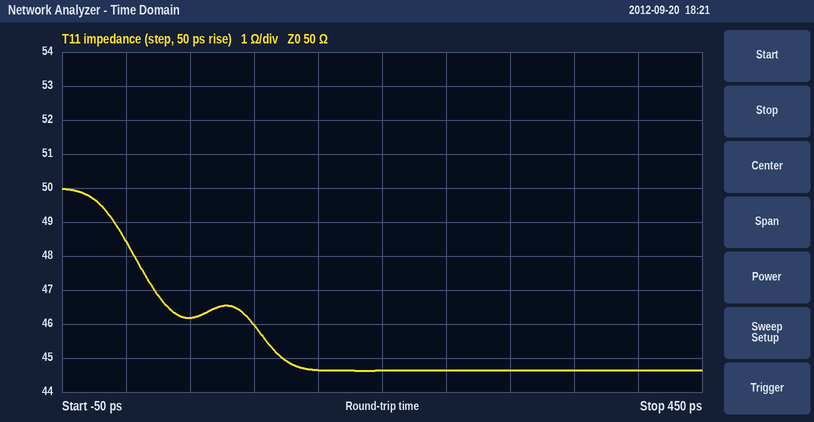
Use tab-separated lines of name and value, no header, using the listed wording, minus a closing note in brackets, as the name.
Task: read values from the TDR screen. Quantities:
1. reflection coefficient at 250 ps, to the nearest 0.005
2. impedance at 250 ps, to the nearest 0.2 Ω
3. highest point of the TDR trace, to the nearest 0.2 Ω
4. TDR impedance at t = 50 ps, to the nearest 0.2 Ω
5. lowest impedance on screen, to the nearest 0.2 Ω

reflection coefficient at 250 ps, to the nearest 0.005	-0.055
impedance at 250 ps, to the nearest 0.2 Ω	44.6 Ω
highest point of the TDR trace, to the nearest 0.2 Ω	50.0 Ω
TDR impedance at t = 50 ps, to the nearest 0.2 Ω	46.2 Ω
lowest impedance on screen, to the nearest 0.2 Ω	44.6 Ω
